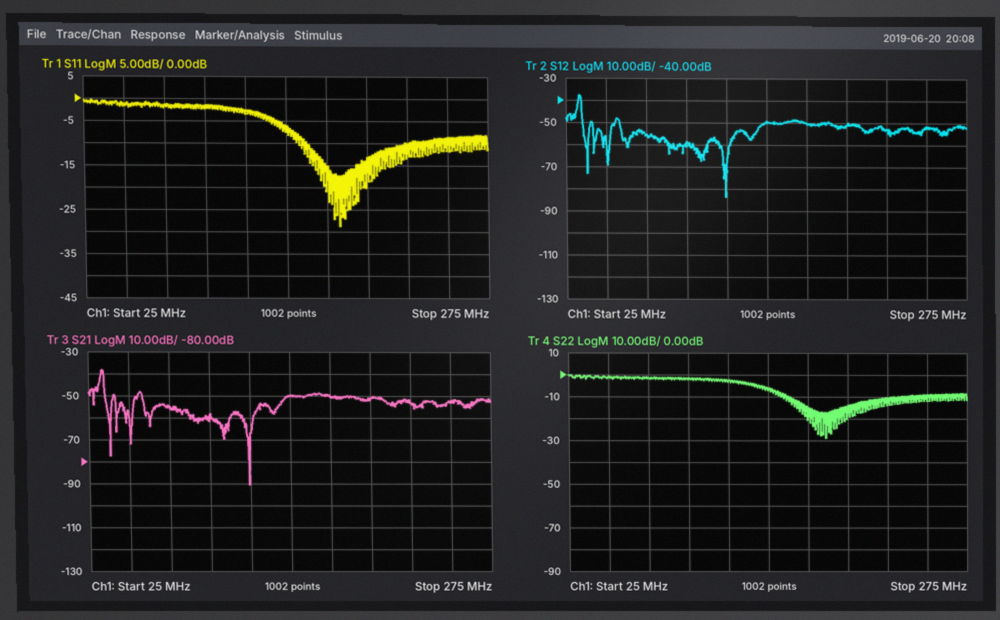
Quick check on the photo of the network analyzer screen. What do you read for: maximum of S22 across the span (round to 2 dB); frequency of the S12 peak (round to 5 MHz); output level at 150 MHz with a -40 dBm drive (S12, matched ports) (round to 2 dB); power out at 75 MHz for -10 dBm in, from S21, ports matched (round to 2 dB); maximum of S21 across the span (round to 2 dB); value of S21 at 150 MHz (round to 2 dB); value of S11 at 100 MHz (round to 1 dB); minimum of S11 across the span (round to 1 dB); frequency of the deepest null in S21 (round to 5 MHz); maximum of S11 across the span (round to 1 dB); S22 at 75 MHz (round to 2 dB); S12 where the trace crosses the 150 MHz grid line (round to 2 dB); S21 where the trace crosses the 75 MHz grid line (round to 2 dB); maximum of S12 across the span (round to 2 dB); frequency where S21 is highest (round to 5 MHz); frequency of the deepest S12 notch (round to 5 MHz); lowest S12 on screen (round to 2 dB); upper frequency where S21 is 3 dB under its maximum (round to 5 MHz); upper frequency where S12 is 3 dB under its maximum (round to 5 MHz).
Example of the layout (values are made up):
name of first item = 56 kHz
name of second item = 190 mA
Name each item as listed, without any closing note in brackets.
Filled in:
maximum of S22 across the span = 0 dB
frequency of the S12 peak = 35 MHz
output level at 150 MHz with a -40 dBm drive (S12, matched ports) = -90 dBm
power out at 75 MHz for -10 dBm in, from S21, ports matched = -66 dBm
maximum of S21 across the span = -38 dB
value of S21 at 150 MHz = -50 dB
value of S11 at 100 MHz = -2 dB
minimum of S11 across the span = -29 dB
frequency of the deepest null in S21 = 125 MHz
maximum of S11 across the span = 0 dB
S22 at 75 MHz = -2 dB
S12 where the trace crosses the 150 MHz grid line = -50 dB
S21 where the trace crosses the 75 MHz grid line = -56 dB
maximum of S12 across the span = -38 dB
frequency where S21 is highest = 35 MHz
frequency of the deepest S12 notch = 125 MHz
lowest S12 on screen = -84 dB
upper frequency where S21 is 3 dB under its maximum = 35 MHz
upper frequency where S12 is 3 dB under its maximum = 35 MHz
